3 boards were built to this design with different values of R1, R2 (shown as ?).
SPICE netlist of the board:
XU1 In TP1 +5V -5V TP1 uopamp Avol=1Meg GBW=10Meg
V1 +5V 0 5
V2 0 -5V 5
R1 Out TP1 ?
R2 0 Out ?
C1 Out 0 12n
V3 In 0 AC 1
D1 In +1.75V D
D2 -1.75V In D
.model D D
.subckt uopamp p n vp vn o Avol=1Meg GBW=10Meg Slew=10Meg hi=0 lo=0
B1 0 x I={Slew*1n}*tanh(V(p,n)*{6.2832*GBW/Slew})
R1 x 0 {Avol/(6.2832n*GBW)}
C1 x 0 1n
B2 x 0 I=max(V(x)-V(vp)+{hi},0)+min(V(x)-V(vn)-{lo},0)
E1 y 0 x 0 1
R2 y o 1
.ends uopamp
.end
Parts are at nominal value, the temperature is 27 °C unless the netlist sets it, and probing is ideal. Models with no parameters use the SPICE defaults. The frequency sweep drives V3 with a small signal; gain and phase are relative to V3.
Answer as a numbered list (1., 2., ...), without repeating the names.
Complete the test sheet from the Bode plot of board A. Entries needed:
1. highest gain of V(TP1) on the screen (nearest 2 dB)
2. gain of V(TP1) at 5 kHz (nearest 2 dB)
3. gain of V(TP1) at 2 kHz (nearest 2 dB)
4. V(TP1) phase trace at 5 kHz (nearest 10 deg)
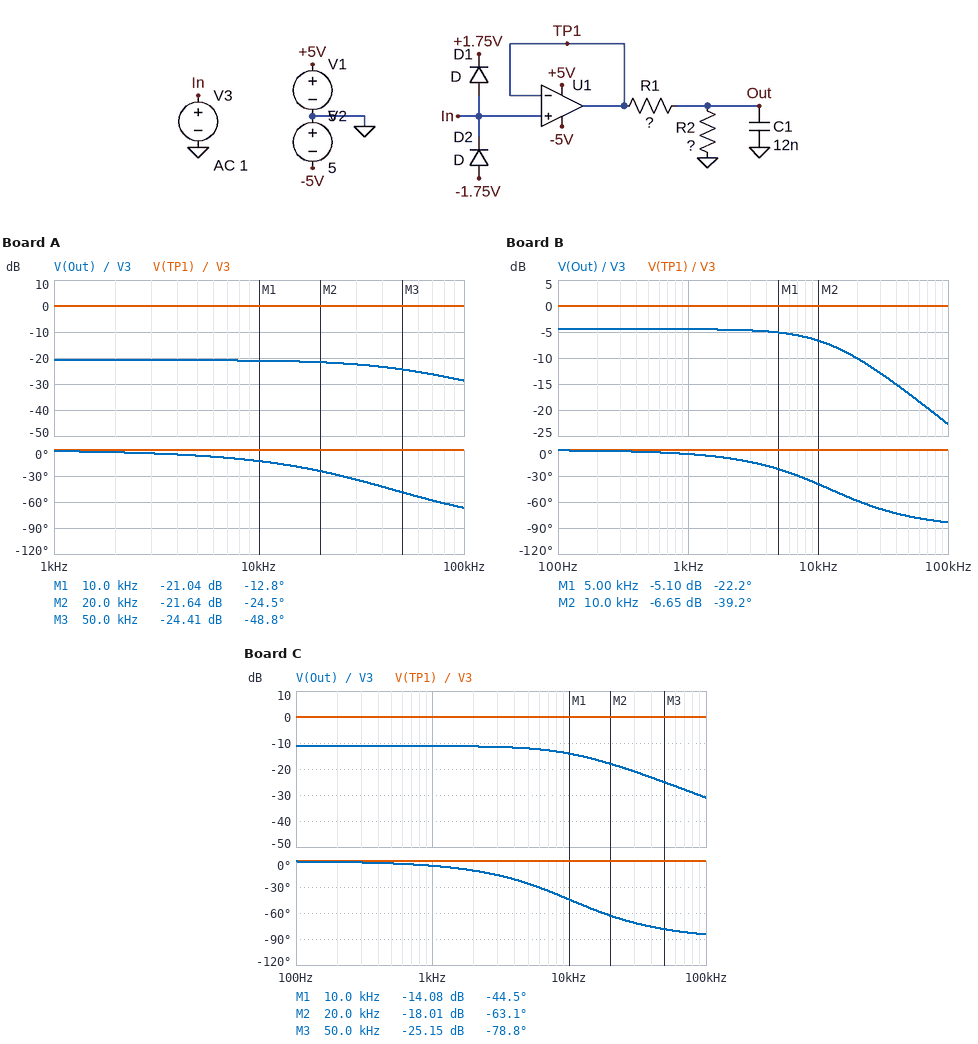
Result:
1. 0 dB
2. 0 dB
3. 0 dB
4. 0 deg
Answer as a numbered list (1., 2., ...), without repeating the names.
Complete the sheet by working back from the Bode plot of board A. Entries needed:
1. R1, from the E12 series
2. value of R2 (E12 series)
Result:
1. 3.3 kΩ
2. 330 Ω
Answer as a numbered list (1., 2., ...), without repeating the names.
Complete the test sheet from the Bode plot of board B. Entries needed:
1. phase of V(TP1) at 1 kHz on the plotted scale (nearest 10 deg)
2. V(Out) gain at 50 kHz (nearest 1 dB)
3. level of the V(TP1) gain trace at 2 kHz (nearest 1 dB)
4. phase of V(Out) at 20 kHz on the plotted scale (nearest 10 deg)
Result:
1. 0 deg
2. -17 dB
3. 0 dB
4. -60 deg
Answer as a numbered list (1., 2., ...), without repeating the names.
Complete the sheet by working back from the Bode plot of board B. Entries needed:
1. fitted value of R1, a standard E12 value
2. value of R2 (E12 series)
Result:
1. 1.8 kΩ
2. 2.7 kΩ
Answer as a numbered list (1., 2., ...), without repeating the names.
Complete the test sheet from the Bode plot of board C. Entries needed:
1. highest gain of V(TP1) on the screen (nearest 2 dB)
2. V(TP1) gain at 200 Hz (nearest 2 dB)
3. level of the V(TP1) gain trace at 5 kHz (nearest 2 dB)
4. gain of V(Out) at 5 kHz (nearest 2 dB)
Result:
1. 0 dB
2. 0 dB
3. 0 dB
4. -12 dB
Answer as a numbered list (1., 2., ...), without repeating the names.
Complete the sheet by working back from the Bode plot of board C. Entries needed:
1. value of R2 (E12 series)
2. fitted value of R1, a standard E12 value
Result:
1. 1.8 kΩ
2. 4.7 kΩ
